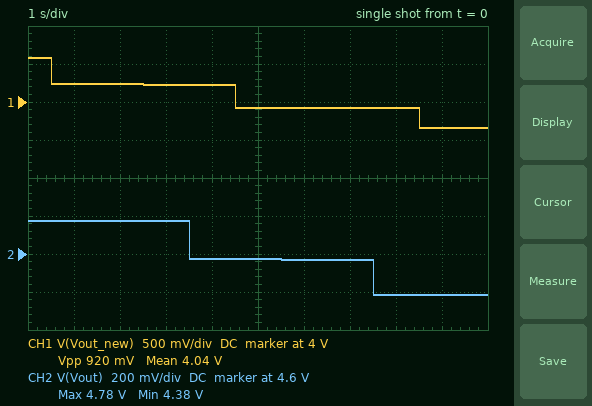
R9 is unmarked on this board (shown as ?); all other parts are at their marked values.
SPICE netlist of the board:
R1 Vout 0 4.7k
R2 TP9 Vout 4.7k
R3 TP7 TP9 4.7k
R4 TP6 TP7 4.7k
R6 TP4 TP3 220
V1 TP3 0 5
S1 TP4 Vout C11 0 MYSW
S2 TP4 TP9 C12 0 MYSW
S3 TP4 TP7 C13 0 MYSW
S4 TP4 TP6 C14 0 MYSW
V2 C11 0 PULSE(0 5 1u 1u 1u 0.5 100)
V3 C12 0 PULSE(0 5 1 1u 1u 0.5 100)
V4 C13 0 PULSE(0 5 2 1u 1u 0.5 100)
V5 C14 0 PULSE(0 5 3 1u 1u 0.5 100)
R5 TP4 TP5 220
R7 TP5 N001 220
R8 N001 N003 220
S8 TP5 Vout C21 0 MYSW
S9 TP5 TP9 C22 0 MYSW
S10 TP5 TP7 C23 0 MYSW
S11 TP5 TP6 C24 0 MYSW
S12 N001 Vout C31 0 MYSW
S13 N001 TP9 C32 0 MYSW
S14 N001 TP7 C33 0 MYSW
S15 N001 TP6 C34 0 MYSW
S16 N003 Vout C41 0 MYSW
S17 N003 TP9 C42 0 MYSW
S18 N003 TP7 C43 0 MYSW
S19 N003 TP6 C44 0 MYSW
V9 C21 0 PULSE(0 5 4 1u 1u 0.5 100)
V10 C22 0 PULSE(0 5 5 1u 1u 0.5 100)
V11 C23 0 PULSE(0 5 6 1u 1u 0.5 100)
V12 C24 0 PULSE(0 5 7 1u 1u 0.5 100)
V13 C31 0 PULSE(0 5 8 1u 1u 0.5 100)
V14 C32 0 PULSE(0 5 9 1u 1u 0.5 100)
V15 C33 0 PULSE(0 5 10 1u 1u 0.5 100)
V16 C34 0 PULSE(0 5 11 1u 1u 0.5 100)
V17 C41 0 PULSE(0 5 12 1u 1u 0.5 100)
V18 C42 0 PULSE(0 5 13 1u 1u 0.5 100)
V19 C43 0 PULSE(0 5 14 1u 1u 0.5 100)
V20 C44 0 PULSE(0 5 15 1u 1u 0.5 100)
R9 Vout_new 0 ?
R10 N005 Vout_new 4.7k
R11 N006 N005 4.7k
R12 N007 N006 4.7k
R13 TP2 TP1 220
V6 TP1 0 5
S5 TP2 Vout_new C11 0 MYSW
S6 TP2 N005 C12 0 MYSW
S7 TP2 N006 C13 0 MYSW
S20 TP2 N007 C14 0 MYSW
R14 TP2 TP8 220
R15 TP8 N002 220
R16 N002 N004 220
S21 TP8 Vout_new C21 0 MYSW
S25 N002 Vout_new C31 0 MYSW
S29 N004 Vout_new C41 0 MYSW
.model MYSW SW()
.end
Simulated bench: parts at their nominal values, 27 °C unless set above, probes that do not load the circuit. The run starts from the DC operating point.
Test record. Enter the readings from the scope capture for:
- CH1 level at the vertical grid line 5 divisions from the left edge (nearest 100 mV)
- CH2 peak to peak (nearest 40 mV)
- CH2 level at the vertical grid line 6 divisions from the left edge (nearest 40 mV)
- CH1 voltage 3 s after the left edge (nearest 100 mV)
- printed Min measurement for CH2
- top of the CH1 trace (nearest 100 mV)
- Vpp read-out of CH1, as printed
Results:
3.9 V
400 mV
4.56 V
4.2 V
4.38 V
4.6 V
920 mV
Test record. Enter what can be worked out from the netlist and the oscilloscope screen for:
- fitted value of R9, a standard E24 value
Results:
2.4 kΩ
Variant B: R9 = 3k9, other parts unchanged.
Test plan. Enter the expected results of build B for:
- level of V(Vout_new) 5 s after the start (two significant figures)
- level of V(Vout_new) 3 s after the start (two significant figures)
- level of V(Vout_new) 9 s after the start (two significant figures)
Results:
4.3 V
4.5 V
4.1 V
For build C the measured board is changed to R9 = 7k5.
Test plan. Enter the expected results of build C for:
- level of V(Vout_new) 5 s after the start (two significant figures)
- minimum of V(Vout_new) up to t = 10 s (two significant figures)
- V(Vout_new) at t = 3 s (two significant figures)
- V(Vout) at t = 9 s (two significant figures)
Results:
4.6 V
4.5 V
4.7 V
4.4 V
